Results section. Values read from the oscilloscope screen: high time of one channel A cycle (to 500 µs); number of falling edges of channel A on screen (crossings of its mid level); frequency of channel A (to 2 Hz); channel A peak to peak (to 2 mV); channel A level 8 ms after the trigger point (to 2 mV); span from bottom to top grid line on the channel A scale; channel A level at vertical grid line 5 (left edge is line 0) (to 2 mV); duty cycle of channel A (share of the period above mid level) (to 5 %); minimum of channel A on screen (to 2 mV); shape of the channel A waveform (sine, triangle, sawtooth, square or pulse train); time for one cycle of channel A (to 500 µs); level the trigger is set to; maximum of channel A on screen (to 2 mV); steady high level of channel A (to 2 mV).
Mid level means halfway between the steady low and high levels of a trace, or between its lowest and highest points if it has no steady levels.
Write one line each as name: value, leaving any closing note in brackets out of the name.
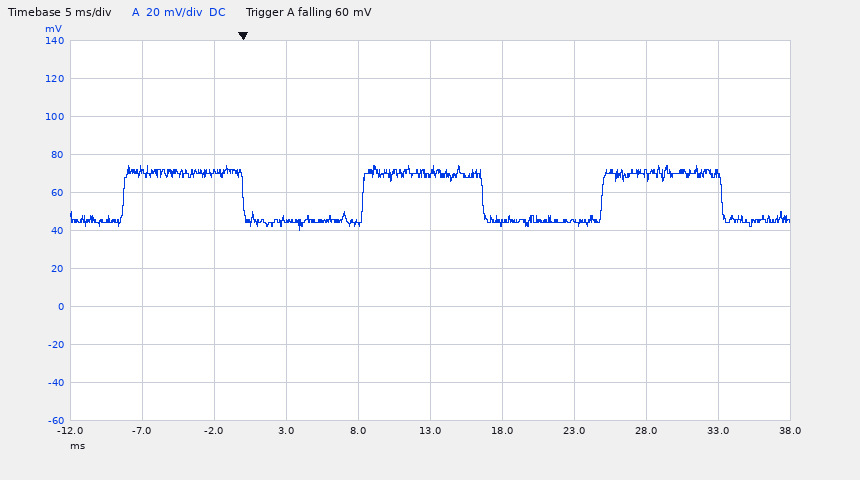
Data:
high time of one channel A cycle: 8.5 ms
number of falling edges of channel A on screen: 3
frequency of channel A: 60 Hz
channel A peak to peak: 34 mV
channel A level 8 ms after the trigger point: 44 mV
span from bottom to top grid line on the channel A scale: 200 mV
channel A level at vertical grid line 5 (left edge is line 0): 70 mV
duty cycle of channel A (share of the period above mid level): 50 %
minimum of channel A on screen: 40 mV
shape of the channel A waveform: square
time for one cycle of channel A: 16.5 ms
level the trigger is set to: 60 mV
maximum of channel A on screen: 74 mV
steady high level of channel A: 70 mV
